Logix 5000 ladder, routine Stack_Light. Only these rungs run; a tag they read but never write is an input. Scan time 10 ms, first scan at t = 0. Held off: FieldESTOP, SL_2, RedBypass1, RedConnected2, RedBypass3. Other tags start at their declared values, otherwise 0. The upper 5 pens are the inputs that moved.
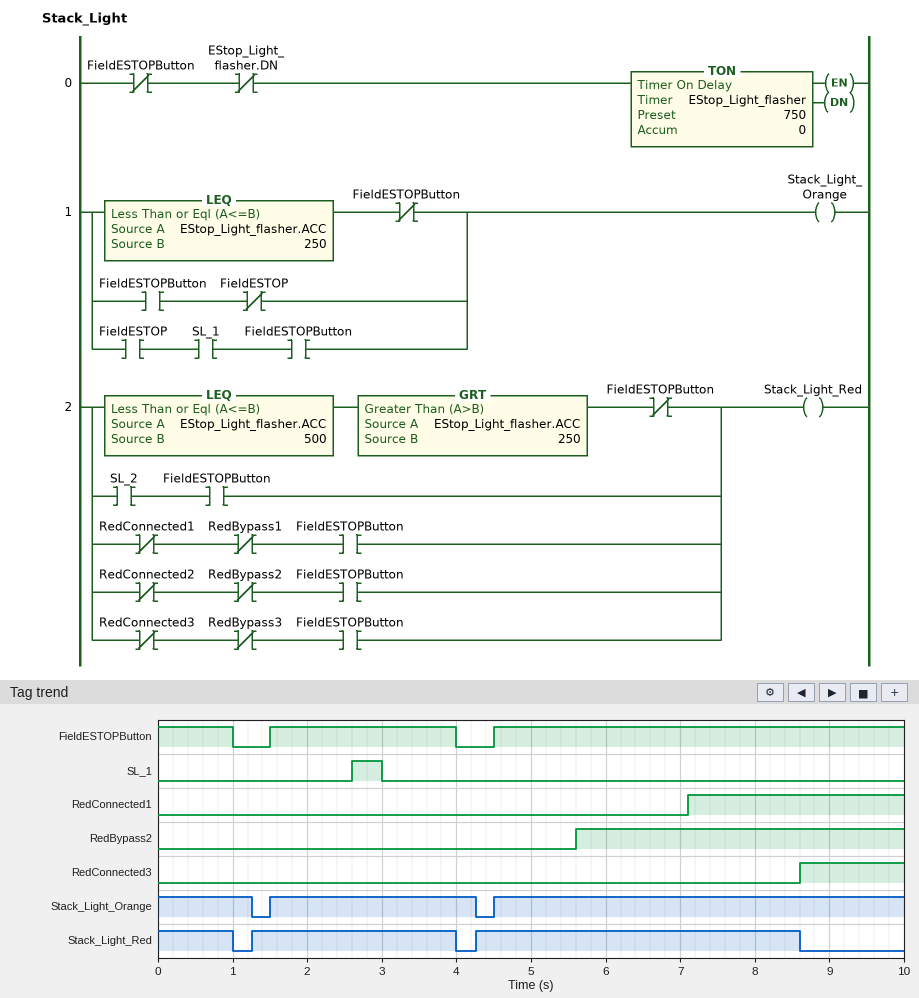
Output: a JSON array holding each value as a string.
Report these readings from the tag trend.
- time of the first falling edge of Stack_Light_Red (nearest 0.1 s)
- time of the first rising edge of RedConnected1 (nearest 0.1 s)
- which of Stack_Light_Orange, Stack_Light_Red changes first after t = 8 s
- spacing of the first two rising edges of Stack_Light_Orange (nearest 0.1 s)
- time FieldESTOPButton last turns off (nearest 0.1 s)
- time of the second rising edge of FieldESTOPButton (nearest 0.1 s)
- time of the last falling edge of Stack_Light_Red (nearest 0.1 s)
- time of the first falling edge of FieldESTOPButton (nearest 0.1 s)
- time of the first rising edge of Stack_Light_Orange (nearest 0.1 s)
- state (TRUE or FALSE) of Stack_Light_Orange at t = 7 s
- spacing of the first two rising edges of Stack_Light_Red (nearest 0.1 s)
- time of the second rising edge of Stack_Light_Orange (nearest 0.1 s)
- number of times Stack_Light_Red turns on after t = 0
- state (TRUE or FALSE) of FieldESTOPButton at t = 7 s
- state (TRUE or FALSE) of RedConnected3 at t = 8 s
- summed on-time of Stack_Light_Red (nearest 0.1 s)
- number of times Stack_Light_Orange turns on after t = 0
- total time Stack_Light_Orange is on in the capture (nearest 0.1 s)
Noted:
["1.0 s", "7.1 s", "Stack_Light_Red", "3.0 s", "4.0 s", "4.5 s", "8.6 s", "1.0 s", "1.5 s", "TRUE", "3.0 s", "4.5 s", "2", "TRUE", "FALSE", "8.1 s", "2", "9.5 s"]
